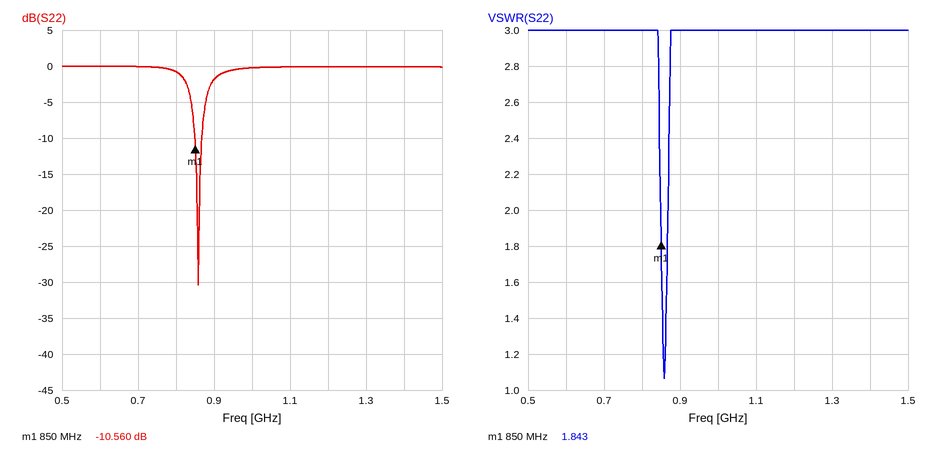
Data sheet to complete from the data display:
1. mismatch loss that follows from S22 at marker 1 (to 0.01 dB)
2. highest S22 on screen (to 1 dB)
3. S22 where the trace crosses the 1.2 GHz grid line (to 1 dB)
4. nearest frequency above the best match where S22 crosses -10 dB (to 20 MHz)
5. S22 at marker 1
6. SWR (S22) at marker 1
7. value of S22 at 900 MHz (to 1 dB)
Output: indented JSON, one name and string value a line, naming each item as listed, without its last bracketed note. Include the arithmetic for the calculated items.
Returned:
{
  "mismatch loss that follows from S22 at marker 1": "−10 log10(1 − 10^(-10.56/10)) ≈ 0.40 dB",
  "highest S22 on screen": "0 dB",
  "S22 where the trace crosses the 1.2 GHz grid line": "0 dB",
  "nearest frequency above the best match where S22 crosses -10 dB": "860 MHz",
  "S22 at marker 1": "-10.560 dB",
  "SWR (S22) at marker 1": "1.843",
  "value of S22 at 900 MHz": "-2 dB"
}
